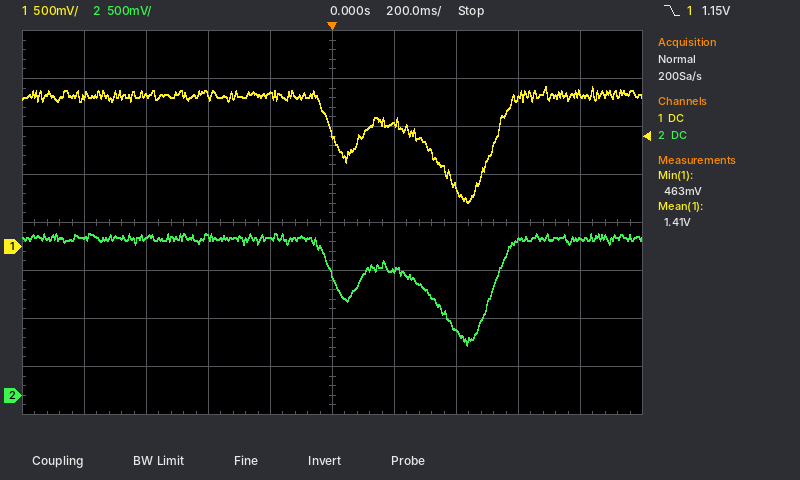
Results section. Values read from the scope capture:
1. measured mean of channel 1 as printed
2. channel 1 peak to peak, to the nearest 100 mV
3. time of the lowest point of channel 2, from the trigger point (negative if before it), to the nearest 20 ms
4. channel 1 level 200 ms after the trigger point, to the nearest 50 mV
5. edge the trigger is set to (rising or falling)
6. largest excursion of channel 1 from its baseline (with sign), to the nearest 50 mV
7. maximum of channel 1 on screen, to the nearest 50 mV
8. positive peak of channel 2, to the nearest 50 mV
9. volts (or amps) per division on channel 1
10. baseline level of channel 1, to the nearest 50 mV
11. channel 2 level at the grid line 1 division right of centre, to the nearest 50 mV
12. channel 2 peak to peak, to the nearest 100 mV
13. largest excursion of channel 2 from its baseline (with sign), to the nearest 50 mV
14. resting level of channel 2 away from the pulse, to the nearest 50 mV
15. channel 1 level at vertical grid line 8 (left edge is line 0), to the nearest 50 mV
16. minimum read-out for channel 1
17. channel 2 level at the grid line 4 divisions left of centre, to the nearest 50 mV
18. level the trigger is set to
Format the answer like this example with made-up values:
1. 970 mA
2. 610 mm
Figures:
1. 1.41 V
2. 1.20 V
3. +440 ms
4. 1.30 V
5. falling
6. -1.10 V
7. 1.65 V
8. 1.70 V
9. 500 mV
10. 1.55 V
11. 1.30 V
12. 1.20 V
13. -1.10 V
14. 1.65 V
15. 1.55 V
16. 463 mV
17. 1.65 V
18. 1.15 V
